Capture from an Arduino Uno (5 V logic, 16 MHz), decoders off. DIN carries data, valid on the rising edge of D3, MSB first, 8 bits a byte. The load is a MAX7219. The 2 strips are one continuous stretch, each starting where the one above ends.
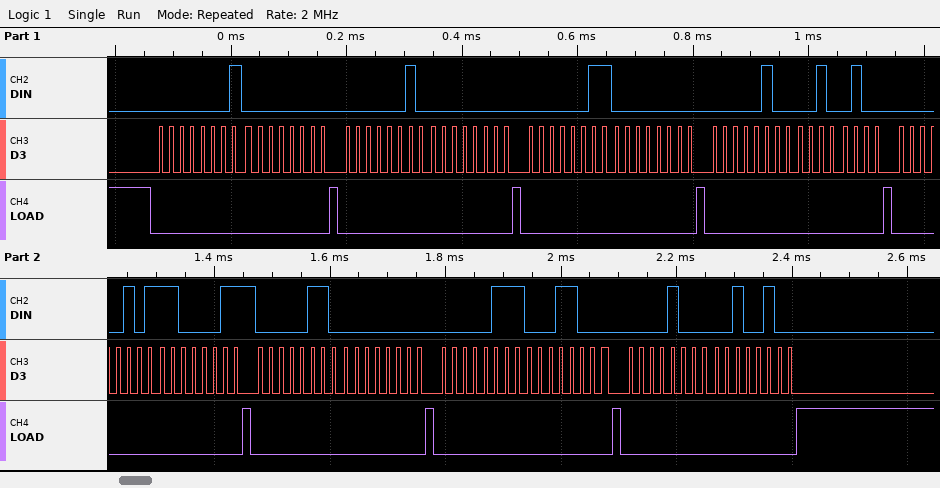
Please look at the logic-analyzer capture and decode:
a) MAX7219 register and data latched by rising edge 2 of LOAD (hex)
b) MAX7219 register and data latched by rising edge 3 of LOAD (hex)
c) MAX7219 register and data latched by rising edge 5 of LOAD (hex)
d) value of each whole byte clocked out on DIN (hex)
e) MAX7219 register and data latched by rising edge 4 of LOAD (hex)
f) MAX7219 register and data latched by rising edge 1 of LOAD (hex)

register 0x2, data 0x00
register 0x3, data 0x00
register 0x5, data 0xC3
0x01 0x00 0x02 0x00 0x03 0x00 0x04 0x24 0x05 0xC3 0x06 0x00 0x07 0x18 0x08 0x24
register 0x4, data 0x24
register 0x1, data 0x00
